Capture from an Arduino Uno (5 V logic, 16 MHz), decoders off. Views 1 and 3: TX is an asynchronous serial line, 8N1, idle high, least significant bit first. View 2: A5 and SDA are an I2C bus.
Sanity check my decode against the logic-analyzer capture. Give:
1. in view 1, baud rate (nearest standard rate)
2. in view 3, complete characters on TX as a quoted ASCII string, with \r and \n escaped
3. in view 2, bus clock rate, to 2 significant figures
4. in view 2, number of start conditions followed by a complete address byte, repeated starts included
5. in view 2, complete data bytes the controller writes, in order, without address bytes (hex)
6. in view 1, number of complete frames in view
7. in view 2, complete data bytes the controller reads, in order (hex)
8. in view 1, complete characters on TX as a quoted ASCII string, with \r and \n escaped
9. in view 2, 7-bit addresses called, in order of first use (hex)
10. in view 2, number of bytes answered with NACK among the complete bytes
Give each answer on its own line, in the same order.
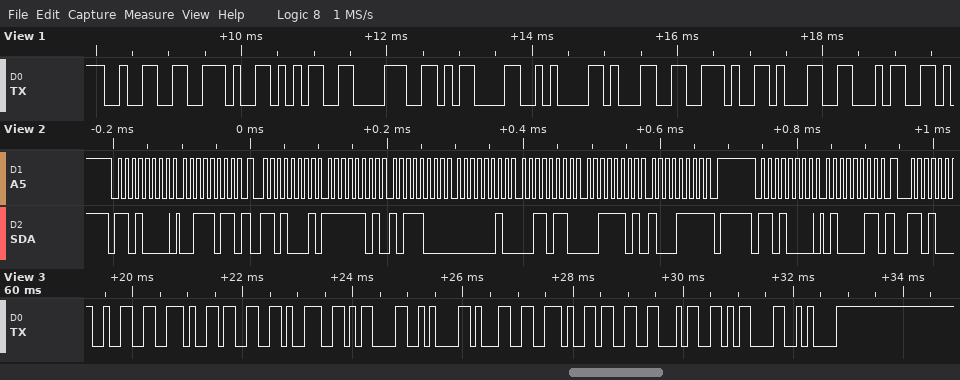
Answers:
9600 baud
"2.39\r\n1.34\r\n"
100 kHz
3
3B 43
10
FD B8 02 36 3D 8F
"2.58\r\n1.14"
0x68
1
